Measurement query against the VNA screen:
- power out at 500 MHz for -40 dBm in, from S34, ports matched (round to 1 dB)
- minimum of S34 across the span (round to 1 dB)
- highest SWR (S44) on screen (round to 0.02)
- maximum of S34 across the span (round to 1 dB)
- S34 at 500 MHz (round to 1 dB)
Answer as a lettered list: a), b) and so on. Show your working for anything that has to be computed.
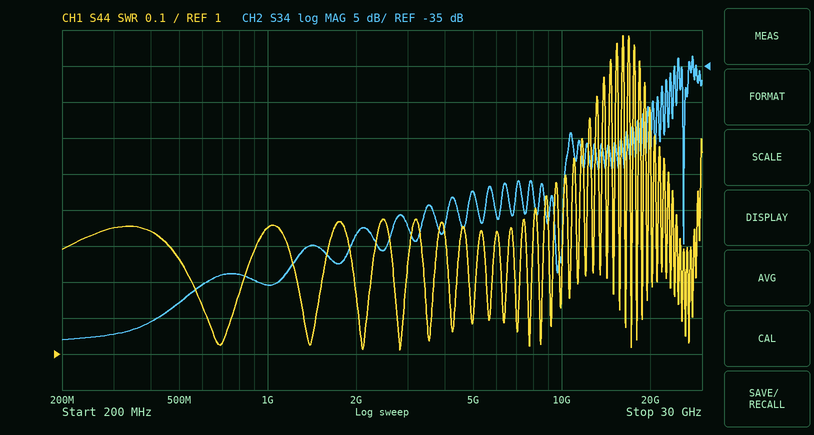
a) -40 dBm + (-68 dB) = -108 dBm
b) -73 dB
c) 1.88
d) -34 dB
e) -68 dB
